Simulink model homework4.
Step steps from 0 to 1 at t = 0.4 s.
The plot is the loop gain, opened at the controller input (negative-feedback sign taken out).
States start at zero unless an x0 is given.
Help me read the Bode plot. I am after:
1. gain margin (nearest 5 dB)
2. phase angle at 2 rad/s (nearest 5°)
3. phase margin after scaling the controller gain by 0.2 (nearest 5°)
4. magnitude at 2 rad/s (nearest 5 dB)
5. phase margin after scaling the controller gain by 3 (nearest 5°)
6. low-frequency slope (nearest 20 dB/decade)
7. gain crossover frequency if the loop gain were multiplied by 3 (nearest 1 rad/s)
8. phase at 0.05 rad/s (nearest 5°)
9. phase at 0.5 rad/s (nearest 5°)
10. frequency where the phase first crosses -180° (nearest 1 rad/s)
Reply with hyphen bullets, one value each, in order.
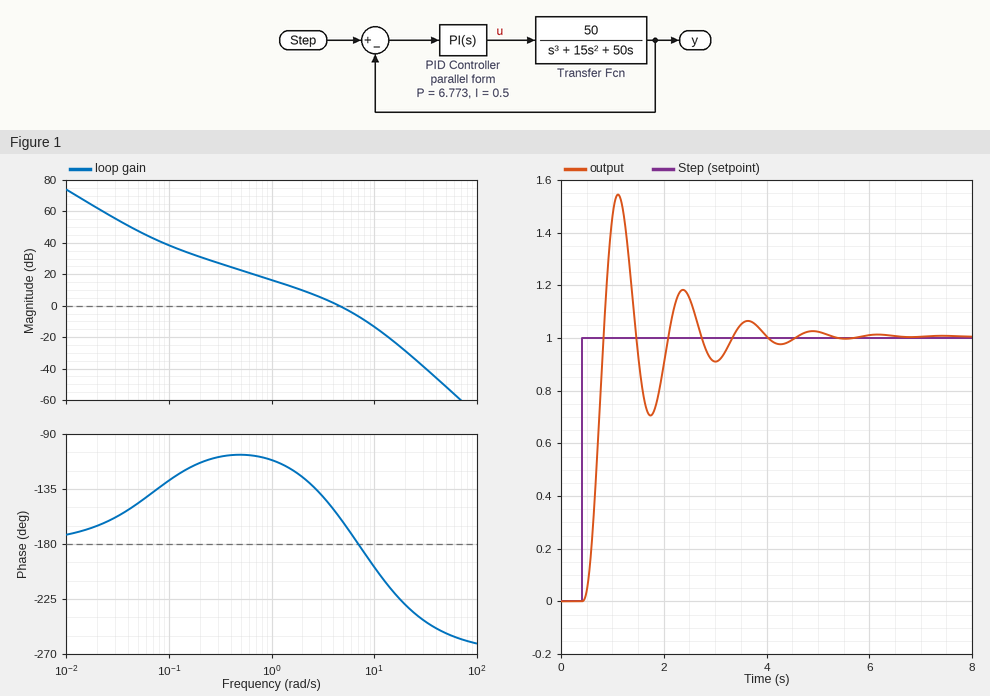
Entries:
- 5 dB
- -125°
- 65°
- 10 dB
- -10°
- -40 dB/decade
- 8 rad/s
- -145°
- -105°
- 7 rad/s
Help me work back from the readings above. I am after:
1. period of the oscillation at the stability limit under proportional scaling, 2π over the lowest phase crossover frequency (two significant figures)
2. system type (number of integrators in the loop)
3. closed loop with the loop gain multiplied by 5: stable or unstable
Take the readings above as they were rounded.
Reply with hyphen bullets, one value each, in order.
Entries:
- 0.90 s
- 2
- unstable
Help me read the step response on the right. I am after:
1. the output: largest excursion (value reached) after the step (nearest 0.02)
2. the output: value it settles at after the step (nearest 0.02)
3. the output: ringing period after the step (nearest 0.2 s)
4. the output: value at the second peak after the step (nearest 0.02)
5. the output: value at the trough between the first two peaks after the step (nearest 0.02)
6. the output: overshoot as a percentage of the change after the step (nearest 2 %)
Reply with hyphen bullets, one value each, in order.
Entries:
- 1.54
- 1.00
- 1.2 s
- 1.18
- 0.70
- 54 %
